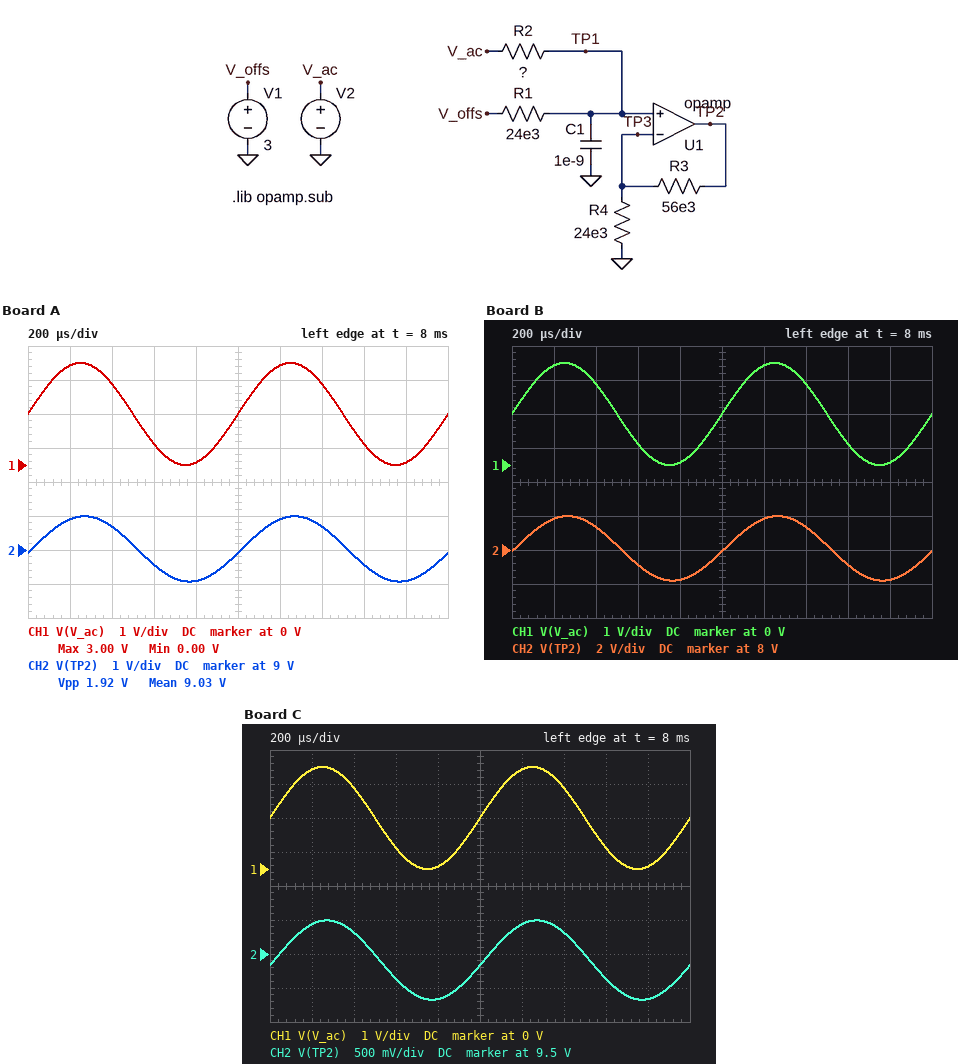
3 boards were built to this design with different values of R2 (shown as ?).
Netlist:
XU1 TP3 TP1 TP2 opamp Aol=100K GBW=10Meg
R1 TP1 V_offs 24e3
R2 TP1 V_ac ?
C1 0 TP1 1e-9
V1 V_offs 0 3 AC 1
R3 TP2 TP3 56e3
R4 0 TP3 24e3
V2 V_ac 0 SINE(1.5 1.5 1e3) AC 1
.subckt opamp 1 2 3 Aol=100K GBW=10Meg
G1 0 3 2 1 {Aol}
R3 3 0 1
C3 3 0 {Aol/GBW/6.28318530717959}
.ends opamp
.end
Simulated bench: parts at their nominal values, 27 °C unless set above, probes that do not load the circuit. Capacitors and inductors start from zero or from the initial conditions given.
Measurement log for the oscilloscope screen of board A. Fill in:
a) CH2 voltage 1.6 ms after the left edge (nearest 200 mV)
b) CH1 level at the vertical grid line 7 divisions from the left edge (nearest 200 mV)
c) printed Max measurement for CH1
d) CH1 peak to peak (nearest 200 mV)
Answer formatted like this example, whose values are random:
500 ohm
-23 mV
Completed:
8.6 V
2.4 V
3.00 V
3.0 V
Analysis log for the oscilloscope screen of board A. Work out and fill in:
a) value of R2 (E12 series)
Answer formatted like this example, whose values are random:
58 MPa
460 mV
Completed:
100 kΩ
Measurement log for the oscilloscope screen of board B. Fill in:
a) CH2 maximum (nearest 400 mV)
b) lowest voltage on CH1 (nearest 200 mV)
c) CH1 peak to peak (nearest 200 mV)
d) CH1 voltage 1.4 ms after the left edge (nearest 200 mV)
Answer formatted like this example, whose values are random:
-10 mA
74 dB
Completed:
10.0 V
0 V
3.0 V
2.4 V
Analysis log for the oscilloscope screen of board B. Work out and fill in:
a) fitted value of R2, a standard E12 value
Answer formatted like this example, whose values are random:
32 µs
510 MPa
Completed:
39 kΩ
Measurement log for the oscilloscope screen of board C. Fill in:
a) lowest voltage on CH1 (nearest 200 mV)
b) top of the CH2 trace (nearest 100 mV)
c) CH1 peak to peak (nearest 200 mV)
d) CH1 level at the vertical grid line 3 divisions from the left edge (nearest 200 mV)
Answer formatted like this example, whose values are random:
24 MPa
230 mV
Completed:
0 V
10.0 V
3.0 V
600 mV
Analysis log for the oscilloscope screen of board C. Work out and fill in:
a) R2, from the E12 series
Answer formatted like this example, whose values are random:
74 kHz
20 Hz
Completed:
180 kΩ
